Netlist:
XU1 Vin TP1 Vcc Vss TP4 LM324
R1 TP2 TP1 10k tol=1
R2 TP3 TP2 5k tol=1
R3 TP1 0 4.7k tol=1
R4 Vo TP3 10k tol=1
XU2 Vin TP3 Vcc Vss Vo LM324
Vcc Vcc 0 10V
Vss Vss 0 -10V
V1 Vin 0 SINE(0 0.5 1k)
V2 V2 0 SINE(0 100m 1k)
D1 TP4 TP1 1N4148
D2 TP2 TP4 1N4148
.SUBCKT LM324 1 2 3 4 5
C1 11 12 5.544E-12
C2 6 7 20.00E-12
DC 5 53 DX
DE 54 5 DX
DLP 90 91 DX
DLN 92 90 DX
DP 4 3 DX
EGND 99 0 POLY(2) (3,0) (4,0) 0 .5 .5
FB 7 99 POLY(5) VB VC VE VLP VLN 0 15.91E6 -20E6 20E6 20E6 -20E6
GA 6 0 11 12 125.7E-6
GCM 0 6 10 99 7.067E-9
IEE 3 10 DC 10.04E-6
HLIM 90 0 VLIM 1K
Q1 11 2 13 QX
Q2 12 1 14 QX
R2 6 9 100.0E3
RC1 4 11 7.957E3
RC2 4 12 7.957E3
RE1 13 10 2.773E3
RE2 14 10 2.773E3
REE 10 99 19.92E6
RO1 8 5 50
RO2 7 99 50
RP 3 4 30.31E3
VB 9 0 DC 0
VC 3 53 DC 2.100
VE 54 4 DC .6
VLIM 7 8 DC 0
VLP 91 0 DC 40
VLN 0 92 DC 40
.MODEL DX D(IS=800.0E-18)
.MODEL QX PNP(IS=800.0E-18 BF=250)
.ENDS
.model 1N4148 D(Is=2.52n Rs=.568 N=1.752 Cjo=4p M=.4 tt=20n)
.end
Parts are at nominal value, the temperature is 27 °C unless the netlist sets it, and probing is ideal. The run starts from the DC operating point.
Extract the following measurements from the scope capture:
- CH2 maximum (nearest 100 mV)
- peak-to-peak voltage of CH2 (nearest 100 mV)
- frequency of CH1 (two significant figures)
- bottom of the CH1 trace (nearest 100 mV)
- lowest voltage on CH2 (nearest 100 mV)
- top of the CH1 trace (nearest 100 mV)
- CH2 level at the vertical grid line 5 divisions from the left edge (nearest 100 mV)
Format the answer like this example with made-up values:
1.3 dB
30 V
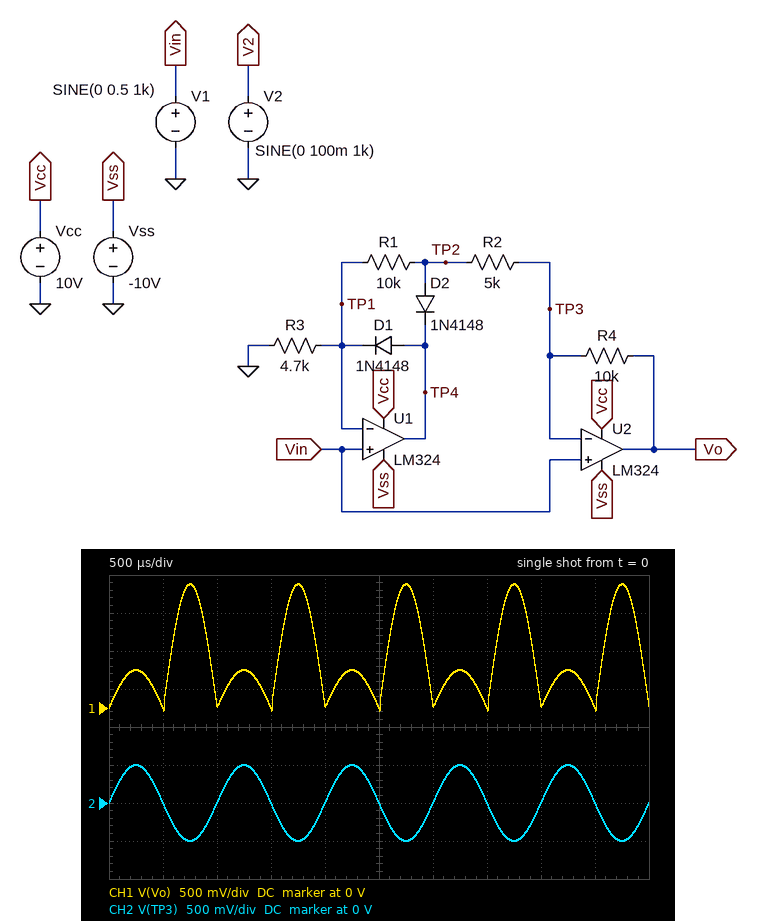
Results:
500 mV
1.0 V
1.0 kHz
0 V
-500 mV
1.6 V
0 V
